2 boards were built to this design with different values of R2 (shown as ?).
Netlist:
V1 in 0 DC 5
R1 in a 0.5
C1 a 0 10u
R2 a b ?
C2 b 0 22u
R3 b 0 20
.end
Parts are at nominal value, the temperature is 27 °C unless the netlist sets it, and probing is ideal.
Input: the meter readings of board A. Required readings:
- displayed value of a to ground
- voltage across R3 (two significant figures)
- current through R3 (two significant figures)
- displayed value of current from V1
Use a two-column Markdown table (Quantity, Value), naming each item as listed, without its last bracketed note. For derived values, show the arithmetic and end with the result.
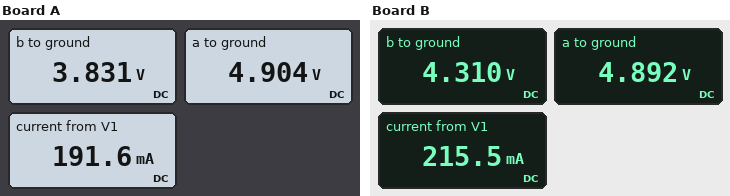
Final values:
| Quantity | Value |
|---|---|
| displayed value of a to ground | 4.904 V |
| voltage across R3 | 3.831 V = 3.8 V |
| current through R3 | (3.831 V) / 20 Ω = 190 mA |
| displayed value of current from V1 | 191.6 mA |
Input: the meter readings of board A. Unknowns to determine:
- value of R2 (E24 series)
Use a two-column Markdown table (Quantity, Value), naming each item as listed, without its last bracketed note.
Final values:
| Quantity | Value |
|---|---|
| value of R2 | 5.6 Ω |
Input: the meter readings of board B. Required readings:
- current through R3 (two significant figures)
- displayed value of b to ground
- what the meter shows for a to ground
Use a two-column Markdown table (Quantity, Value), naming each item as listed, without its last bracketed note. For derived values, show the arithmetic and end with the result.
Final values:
| Quantity | Value |
|---|---|
| current through R3 | (4.31 V) / 20 Ω = 220 mA |
| displayed value of b to ground | 4.310 V |
| what the meter shows for a to ground | 4.892 V |
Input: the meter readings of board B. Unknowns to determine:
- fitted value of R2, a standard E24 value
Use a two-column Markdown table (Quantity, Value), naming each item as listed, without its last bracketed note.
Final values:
| Quantity | Value |
|---|---|
| fitted value of R2, a standard E24 value | 2.7 Ω |
